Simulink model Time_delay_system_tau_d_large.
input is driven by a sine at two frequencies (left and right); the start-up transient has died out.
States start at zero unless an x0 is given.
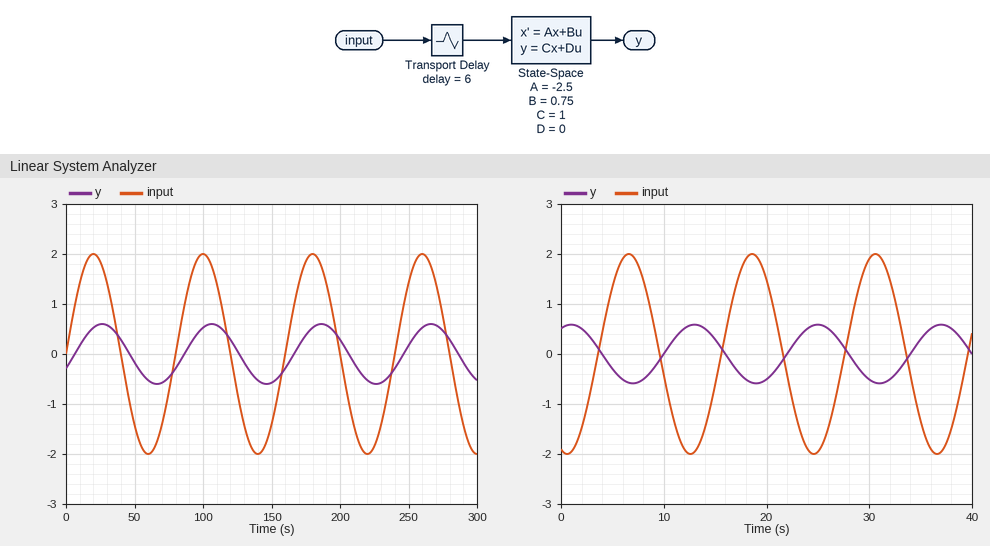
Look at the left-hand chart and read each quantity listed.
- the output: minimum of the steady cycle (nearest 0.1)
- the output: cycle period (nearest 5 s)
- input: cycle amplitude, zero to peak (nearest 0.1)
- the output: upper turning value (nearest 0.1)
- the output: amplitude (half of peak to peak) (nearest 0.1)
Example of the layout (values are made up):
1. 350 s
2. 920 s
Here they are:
1. -0.6
2. 80 s
3. 2.0
4. 0.6
5. 0.6
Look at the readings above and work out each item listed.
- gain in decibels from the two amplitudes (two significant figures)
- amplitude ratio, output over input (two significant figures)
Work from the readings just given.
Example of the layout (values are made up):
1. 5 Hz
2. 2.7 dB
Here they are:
1. -10 dB
2. 0.30
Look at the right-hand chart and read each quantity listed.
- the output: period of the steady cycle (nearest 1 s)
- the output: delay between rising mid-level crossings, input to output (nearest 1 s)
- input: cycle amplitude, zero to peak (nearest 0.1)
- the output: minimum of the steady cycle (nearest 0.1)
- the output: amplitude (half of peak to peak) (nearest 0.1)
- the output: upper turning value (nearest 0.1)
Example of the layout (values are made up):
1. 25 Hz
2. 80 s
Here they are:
1. 12 s
2. 6 s
3. 2.0
4. -0.6
5. 0.6
6. 0.6
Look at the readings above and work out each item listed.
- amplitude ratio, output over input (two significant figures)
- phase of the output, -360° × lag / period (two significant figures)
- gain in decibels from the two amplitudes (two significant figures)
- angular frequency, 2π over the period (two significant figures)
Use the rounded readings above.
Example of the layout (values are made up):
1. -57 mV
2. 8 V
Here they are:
1. 0.30
2. -180°
3. -10 dB
4. 0.52 rad/s
